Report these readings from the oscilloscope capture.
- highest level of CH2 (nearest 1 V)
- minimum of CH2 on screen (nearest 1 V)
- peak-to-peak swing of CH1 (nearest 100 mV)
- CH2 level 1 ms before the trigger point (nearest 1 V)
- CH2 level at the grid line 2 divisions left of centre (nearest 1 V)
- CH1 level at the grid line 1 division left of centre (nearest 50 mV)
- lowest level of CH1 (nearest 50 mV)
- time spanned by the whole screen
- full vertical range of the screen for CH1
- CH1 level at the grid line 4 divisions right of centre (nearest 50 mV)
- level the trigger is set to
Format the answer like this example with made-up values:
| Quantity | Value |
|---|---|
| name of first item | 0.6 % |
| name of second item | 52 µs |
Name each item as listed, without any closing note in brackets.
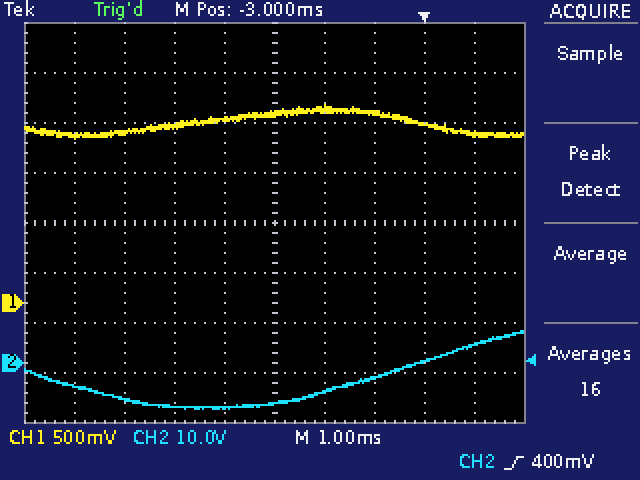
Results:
| Quantity | Value |
|---|---|
| highest level of CH2 | 6 V |
| minimum of CH2 on screen | -9 V |
| peak-to-peak swing of CH1 | 300 mV |
| CH2 level 1 ms before the trigger point | -3 V |
| CH2 level at the grid line 2 divisions left of centre | -9 V |
| CH1 level at the grid line 1 division left of centre | 1.85 V |
| lowest level of CH1 | 1.65 V |
| time spanned by the whole screen | 10 ms |
| full vertical range of the screen for CH1 | 4 V |
| CH1 level at the grid line 4 divisions right of centre | 1.70 V |
| level the trigger is set to | 400 mV |
